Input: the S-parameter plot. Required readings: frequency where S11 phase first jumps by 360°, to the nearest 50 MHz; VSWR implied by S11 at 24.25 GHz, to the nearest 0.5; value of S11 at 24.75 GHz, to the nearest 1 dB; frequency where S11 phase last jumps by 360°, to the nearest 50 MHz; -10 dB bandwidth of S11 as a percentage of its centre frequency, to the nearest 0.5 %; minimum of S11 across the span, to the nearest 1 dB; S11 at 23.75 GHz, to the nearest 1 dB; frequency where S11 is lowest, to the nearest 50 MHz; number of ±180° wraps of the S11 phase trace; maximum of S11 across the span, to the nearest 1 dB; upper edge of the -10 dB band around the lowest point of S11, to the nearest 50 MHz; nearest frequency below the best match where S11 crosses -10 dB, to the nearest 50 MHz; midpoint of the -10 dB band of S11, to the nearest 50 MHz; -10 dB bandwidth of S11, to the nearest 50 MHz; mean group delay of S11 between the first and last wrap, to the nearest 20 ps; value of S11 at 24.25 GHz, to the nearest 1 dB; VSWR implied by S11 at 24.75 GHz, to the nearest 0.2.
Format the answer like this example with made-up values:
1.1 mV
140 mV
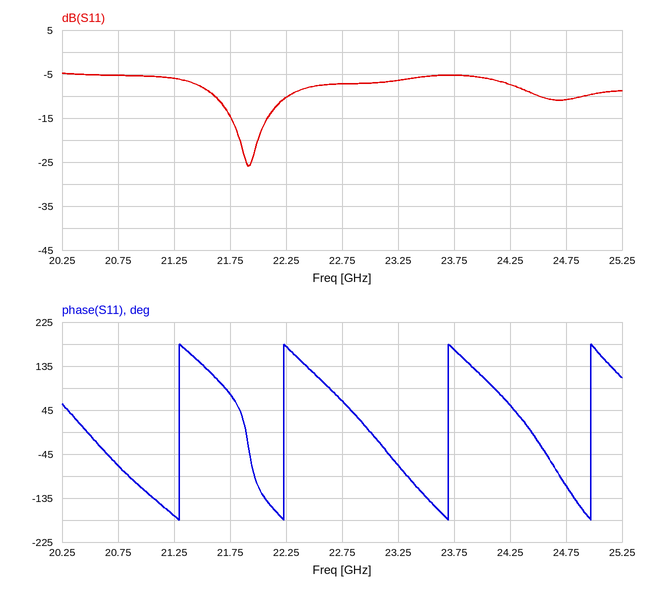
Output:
21.30 GHz
2.5
-11 dB
24.95 GHz
3.0 %
-26 dB
-5 dB
21.90 GHz
4
-5 dB
22.25 GHz
21.60 GHz
21.95 GHz
650 MHz
820 ps
-7 dB
1.8
